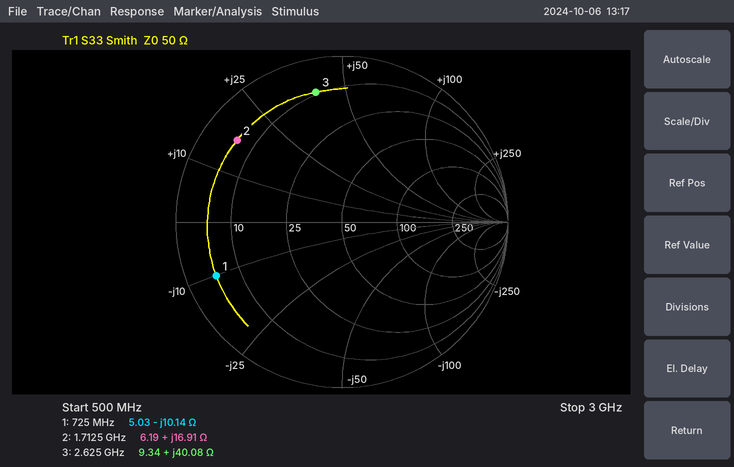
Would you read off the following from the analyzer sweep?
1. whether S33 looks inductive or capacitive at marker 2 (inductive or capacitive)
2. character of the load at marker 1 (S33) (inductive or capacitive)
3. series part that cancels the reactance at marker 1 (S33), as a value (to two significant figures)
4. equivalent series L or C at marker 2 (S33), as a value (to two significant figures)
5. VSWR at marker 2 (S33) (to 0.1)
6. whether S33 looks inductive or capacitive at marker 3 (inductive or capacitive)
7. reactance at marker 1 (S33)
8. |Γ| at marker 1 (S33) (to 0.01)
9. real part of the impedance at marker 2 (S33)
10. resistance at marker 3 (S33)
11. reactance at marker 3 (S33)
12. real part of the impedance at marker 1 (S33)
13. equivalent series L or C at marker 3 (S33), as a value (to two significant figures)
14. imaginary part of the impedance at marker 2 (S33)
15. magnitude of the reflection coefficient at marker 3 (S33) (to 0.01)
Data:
inductive
capacitive
2.2 nH
1.6 nH
9.0
inductive
-10.14 Ω
0.82
6.19 Ω
9.34 Ω
+40.08 Ω
5.03 Ω
2.4 nH
+16.91 Ω
0.80
